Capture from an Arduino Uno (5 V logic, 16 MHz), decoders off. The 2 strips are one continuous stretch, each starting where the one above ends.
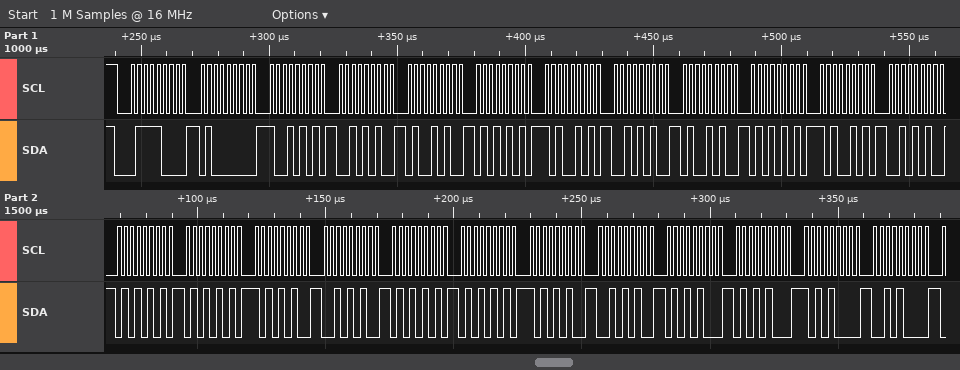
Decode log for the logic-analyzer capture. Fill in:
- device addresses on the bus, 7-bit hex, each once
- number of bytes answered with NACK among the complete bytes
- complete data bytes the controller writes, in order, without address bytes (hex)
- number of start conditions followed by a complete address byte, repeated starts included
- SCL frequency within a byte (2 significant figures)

0x3C
0
40 95 2A 4A 55 A5 2A 4A 55 A5 2A 55 55 AA 2A 55 55 AA 2A 54 54 A8 28
1
400 kHz
